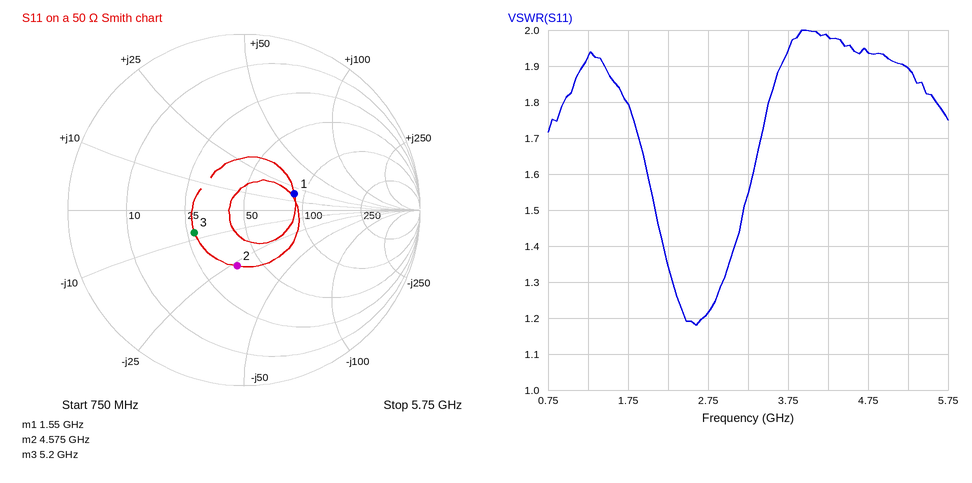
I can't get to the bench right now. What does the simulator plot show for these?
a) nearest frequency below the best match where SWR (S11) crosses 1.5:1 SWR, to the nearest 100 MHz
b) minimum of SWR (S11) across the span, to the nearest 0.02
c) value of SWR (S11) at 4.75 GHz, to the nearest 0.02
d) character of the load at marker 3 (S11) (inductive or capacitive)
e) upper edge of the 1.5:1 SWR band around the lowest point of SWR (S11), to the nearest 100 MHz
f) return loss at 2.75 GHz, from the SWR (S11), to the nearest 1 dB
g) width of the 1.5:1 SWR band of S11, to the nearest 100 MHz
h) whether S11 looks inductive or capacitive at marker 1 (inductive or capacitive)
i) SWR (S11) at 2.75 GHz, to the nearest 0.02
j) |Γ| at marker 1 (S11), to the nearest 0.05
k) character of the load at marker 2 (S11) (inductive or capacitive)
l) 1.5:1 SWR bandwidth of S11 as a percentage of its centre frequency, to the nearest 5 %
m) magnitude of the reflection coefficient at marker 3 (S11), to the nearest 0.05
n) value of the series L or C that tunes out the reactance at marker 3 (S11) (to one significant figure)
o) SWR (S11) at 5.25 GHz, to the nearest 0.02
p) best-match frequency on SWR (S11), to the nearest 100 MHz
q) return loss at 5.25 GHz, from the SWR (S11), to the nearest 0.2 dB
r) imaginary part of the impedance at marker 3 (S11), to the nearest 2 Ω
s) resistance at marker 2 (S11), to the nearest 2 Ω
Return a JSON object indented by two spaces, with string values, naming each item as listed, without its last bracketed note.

{
  "nearest frequency below the best match where SWR (S11) crosses 1.5:1 SWR, to the nearest 100 MHz": "2.1 GHz",
  "minimum of SWR (S11) across the span, to the nearest 0.02": "1.18",
  "value of SWR (S11) at 4.75 GHz, to the nearest 0.02": "1.94",
  "character of the load at marker 3 (S11)": "capacitive",
  "upper edge of the 1.5:1 SWR band around the lowest point of SWR (S11), to the nearest 100 MHz": "3.2 GHz",
  "return loss at 2.75 GHz, from the SWR (S11), to the nearest 1 dB": "20 dB",
  "width of the 1.5:1 SWR band of S11, to the nearest 100 MHz": "1.1 GHz",
  "whether S11 looks inductive or capacitive at marker 1": "inductive",
  "SWR (S11) at 2.75 GHz, to the nearest 0.02": "1.22",
  "|Γ| at marker 1 (S11), to the nearest 0.05": "0.30",
  "character of the load at marker 2 (S11)": "capacitive",
  "1.5:1 SWR bandwidth of S11 as a percentage of its centre frequency, to the nearest 5 %": "40 %",
  "magnitude of the reflection coefficient at marker 3 (S11), to the nearest 0.05": "0.30",
  "value of the series L or C that tunes out the reactance at marker 3 (S11)": "200 pH",
  "SWR (S11) at 5.25 GHz, to the nearest 0.02": "1.90",
  "best-match frequency on SWR (S11), to the nearest 100 MHz": "2.6 GHz",
  "return loss at 5.25 GHz, from the SWR (S11), to the nearest 0.2 dB": "10.2 dB",
  "imaginary part of the impedance at marker 3 (S11), to the nearest 2 Ω": "-8 Ω",
  "resistance at marker 2 (S11), to the nearest 2 Ω": "38 Ω"
}
